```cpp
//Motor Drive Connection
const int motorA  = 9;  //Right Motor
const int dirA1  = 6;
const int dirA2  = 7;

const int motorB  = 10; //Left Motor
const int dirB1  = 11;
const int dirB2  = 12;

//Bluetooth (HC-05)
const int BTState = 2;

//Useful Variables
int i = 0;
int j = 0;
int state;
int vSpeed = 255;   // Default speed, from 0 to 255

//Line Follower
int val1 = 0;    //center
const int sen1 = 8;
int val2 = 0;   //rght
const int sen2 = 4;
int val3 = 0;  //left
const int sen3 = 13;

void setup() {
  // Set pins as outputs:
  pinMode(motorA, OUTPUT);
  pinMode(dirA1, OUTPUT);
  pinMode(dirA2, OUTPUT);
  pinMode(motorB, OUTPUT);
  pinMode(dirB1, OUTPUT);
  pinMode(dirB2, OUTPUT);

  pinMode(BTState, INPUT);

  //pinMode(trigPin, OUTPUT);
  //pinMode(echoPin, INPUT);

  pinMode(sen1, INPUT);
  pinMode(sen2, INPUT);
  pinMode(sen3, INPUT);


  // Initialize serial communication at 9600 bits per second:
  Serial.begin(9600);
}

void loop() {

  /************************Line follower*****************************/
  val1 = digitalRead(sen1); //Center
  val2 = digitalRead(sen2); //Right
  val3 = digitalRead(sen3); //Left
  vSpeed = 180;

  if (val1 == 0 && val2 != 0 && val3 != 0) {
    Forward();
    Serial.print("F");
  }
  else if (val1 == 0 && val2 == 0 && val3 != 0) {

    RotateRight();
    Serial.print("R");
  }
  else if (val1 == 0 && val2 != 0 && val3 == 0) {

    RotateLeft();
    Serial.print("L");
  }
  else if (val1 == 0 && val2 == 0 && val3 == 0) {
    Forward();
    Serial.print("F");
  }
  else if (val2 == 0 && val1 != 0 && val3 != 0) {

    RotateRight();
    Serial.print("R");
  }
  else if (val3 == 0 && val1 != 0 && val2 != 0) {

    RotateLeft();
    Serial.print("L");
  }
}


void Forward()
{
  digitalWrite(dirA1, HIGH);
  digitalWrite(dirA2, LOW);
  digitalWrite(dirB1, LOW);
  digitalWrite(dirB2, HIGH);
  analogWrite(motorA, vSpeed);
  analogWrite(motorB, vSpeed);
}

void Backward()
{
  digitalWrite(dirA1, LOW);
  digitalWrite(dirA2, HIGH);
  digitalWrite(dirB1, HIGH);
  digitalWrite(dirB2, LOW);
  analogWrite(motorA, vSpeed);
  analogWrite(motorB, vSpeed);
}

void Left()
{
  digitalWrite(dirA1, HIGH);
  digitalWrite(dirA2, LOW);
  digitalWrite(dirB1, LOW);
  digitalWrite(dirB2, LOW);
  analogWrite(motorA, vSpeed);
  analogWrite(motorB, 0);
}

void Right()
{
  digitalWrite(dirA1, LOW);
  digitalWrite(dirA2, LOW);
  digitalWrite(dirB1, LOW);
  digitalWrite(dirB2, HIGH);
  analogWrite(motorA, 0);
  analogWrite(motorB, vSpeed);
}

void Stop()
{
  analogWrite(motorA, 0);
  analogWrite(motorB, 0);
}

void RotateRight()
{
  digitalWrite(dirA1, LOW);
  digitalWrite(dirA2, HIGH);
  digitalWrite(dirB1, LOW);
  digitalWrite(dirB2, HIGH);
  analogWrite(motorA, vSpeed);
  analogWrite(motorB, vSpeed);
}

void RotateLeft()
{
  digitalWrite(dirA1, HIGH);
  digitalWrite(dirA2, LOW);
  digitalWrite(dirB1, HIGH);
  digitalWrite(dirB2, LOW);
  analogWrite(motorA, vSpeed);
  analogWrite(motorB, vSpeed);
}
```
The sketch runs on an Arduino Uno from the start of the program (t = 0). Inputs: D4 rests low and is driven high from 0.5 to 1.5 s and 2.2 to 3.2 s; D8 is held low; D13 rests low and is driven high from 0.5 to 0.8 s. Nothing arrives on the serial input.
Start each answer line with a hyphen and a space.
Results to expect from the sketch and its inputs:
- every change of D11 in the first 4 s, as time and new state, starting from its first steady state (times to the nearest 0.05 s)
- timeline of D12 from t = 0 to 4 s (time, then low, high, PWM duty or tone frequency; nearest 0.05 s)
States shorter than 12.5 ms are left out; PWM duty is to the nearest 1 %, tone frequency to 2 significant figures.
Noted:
- 0 s low; 0.8 s high; 1.5 s low; 2.2 s high; 3.2 s low
- 0 s high; 0.8 s low; 1.5 s high; 2.2 s low; 3.2 s high
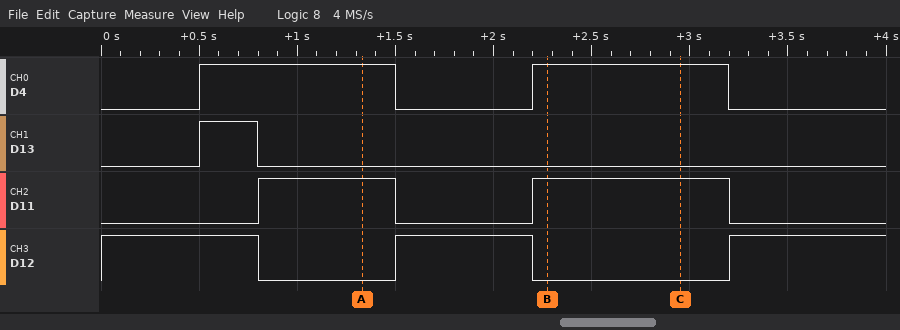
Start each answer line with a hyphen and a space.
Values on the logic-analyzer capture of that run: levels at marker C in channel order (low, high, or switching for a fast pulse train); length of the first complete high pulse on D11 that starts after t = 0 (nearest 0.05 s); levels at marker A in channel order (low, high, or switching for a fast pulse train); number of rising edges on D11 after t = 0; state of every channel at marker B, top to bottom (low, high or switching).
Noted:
- D4 high, D13 low, D11 high, D12 low
- 0.70 s
- D4 high, D13 low, D11 high, D12 low
- 2
- D4 high, D13 low, D11 high, D12 low
